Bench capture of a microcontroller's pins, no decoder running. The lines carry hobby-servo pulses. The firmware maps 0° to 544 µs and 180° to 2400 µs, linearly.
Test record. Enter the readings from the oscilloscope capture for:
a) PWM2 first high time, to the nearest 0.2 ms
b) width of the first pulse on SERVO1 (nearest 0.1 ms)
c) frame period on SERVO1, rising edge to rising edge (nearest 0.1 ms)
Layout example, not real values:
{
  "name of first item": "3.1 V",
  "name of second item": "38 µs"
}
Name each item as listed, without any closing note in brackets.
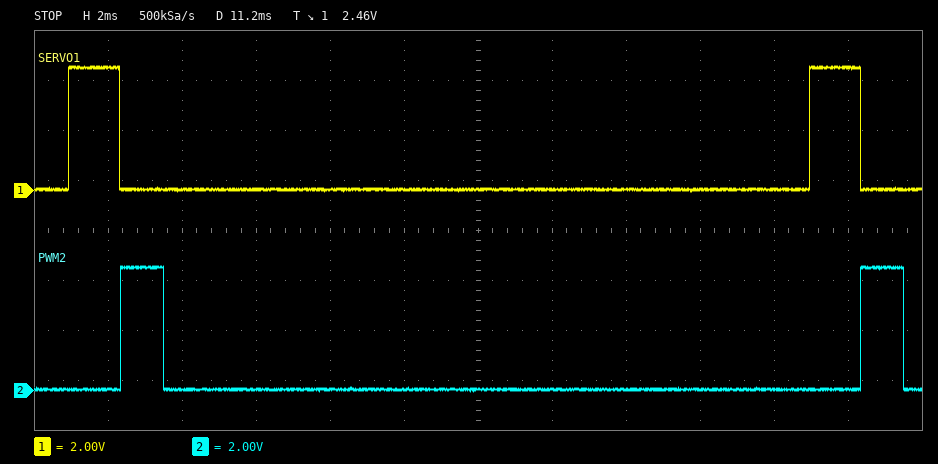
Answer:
{
  "PWM2 first high time, to the nearest 0.2 ms": "1.2 ms",
  "width of the first pulse on SERVO1": "1.4 ms",
  "frame period on SERVO1, rising edge to rising edge": "20.0 ms"
}
